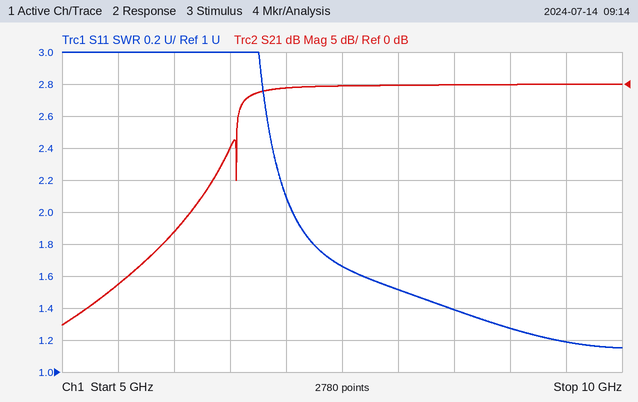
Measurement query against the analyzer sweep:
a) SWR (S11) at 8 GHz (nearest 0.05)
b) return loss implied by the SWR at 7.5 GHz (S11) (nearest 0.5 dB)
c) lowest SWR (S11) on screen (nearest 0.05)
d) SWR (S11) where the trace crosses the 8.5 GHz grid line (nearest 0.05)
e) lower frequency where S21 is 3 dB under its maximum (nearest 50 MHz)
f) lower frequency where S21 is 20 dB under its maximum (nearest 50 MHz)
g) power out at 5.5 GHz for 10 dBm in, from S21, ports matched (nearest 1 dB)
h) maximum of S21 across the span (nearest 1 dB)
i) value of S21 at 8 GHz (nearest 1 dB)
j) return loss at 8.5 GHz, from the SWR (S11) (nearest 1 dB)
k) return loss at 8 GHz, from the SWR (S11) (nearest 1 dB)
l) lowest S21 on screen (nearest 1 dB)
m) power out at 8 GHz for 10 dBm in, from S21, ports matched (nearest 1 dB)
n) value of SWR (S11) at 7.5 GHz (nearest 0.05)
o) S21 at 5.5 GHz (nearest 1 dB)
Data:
1.50
12.0 dB
1.15
1.40
6.60 GHz
6.15 GHz
-21 dBm
0 dB
0 dB
16 dB
14 dB
-38 dB
10 dBm
1.65
-31 dB
